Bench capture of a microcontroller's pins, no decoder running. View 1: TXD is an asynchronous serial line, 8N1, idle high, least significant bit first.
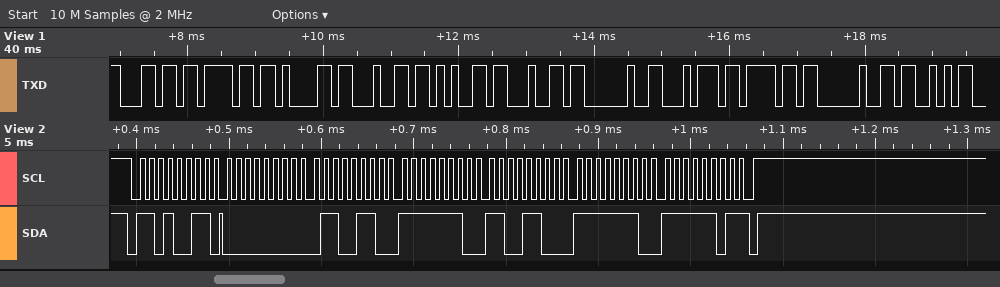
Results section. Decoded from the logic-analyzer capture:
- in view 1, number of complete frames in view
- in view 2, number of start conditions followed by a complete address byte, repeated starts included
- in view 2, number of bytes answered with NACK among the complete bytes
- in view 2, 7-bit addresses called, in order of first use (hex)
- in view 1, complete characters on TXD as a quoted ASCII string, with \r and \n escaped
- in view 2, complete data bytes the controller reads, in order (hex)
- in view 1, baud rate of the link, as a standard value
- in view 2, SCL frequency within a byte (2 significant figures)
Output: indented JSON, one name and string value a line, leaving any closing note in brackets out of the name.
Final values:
{
  "in view 1, number of complete frames in view": "11",
  "in view 2, number of start conditions followed by a complete address byte, repeated starts included": "1",
  "in view 2, number of bytes answered with NACK among the complete bytes": "1",
  "in view 2, 7-bit addresses called, in order of first use": "0x69",
  "in view 1, complete characters on TXD as a quoted ASCII string, with \\r and \\n escaped": "\"loaded to S\"",
  "in view 2, complete data bytes the controller reads, in order": "00 66 FE CC FE FD",
  "in view 1, baud rate of the link, as a standard value": "9600 baud",
  "in view 2, SCL frequency within a byte": "100 kHz"
}
